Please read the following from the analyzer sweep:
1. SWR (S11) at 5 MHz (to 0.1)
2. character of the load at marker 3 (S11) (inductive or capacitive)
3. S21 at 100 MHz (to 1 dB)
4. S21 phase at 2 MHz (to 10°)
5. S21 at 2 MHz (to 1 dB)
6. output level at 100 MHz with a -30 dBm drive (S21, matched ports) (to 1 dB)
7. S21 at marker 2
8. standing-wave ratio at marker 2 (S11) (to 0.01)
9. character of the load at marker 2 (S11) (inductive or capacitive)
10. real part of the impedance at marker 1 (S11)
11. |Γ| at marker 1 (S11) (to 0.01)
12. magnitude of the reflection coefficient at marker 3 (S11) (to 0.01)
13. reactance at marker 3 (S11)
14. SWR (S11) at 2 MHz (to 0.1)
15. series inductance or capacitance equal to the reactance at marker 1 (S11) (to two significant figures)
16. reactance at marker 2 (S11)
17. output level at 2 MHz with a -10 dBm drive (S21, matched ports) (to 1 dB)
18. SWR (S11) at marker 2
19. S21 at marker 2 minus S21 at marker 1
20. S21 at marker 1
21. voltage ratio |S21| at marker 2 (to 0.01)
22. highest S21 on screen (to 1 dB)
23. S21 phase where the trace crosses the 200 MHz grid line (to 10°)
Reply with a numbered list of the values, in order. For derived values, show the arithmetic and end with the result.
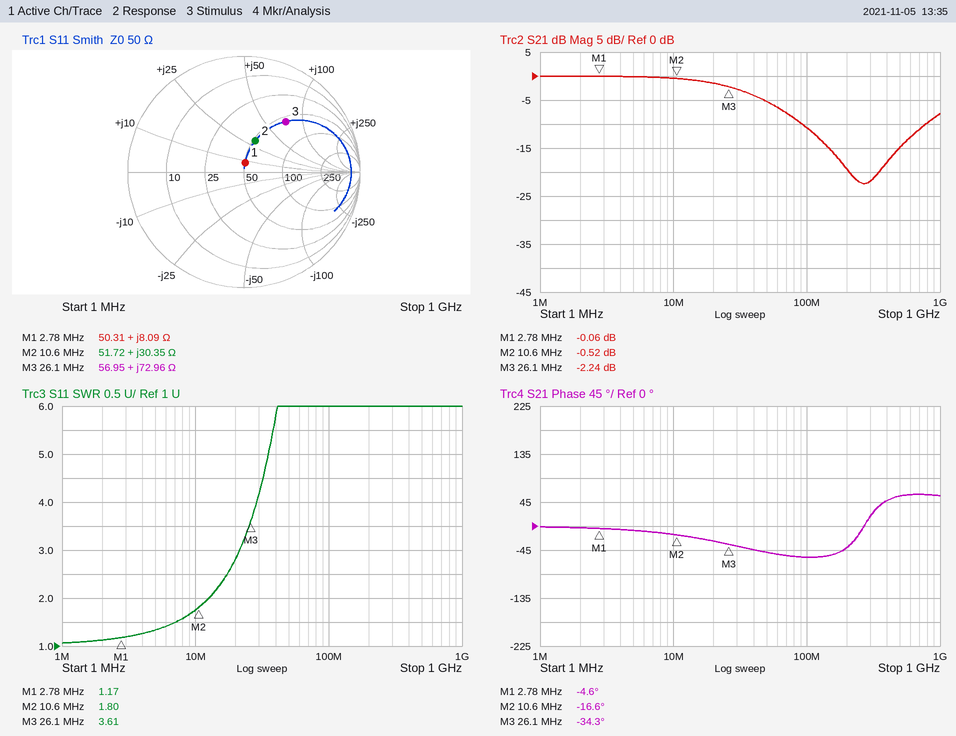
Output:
1. 1.3
2. inductive
3. -11 dB
4. 0°
5. 0 dB
6. -30 dBm + (-11 dB) = -41 dBm
7. -0.52 dB
8. 1.80
9. inductive
10. 50.31 Ω
11. 0.08
12. 0.57
13. +72.96 Ω
14. 1.1
15. L = 8.09 Ω/(2π × 2.78 MHz) ≈ 463 nH, so 460 nH to two significant figures
16. +30.35 Ω
17. -10 dBm + (0 dB) = -10 dBm
18. 1.80
19. -0.52 − (-0.06) = -0.46 dB
20. -0.06 dB
21. 10^(-0.52/20) ≈ 0.94
22. 0 dB
23. -40°
